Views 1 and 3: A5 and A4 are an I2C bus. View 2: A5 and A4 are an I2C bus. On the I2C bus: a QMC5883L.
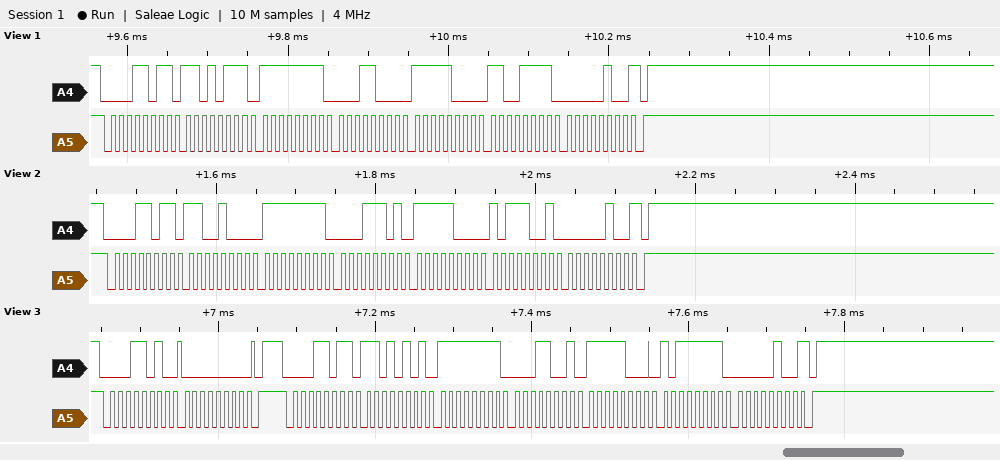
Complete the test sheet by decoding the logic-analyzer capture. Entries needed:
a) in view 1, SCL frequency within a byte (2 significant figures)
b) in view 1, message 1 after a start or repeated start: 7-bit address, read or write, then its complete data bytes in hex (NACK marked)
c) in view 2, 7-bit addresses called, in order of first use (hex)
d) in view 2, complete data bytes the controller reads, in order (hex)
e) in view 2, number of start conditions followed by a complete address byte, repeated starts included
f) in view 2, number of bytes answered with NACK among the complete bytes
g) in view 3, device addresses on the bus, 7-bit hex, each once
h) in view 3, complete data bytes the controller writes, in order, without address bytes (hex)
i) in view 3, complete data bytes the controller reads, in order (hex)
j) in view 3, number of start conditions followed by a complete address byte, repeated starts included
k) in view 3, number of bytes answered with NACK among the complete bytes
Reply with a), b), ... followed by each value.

a) 100 kHz
b) 0x0D read: D7 FF 18 F8 CF 04 NACK
c) 0x0D
d) C8 FF 1D F8 B9 04
e) 1
f) 1
g) 0x0D
h) 00
i) D5 FF 19 F8 BF 04
j) 2
k) 1
